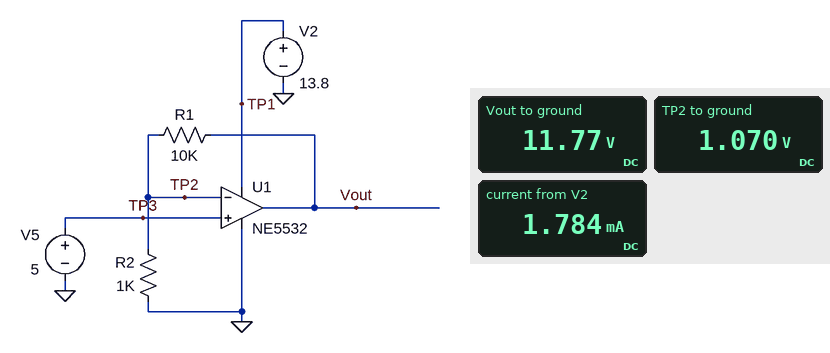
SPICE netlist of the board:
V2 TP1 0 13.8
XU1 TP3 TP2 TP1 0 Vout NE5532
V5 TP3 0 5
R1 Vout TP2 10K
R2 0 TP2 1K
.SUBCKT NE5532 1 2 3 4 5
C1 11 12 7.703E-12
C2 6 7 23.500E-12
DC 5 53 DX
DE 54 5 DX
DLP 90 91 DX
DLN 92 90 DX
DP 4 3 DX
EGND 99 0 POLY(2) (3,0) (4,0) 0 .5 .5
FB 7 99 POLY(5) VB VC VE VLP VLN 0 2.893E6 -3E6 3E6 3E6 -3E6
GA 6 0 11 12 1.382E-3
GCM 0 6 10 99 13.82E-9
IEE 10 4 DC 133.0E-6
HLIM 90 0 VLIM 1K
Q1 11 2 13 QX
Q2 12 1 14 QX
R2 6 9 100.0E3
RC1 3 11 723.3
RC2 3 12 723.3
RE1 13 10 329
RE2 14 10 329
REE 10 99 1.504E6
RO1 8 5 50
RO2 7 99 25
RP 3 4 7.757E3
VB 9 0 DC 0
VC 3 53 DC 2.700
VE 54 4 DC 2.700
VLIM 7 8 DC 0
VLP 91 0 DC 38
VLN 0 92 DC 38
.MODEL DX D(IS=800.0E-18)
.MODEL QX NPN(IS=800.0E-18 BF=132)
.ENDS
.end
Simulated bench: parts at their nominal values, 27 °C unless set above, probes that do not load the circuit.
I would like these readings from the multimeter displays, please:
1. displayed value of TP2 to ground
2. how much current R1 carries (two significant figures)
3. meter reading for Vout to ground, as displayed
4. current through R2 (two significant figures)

1.070 V
1.1 mA
11.77 V
1.1 mA
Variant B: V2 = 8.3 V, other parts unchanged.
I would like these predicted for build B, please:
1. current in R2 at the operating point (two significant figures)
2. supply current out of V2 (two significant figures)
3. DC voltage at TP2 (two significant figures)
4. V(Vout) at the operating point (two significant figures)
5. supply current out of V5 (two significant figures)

570 µA
1.1 mA
570 mV
6.3 V
1.0 µA
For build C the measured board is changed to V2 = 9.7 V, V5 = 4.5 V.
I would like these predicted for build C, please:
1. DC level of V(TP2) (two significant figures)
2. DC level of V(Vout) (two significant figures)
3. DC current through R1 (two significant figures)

700 mV
7.7 V
700 µA
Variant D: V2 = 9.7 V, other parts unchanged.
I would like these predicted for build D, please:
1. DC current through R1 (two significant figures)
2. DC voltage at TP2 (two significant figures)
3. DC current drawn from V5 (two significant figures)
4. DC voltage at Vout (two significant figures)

700 µA
700 mV
1.0 µA
7.7 V
